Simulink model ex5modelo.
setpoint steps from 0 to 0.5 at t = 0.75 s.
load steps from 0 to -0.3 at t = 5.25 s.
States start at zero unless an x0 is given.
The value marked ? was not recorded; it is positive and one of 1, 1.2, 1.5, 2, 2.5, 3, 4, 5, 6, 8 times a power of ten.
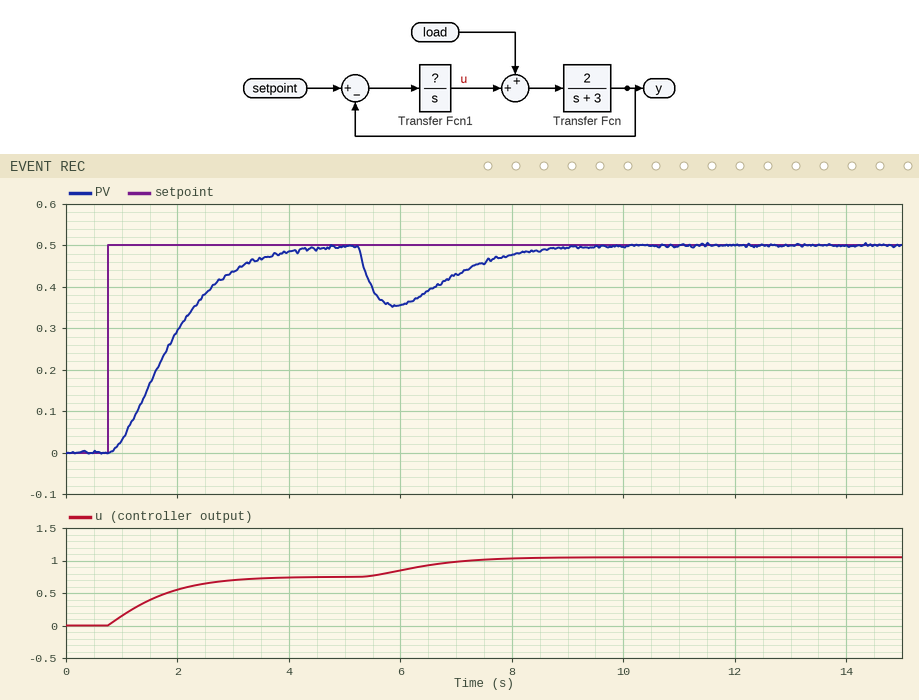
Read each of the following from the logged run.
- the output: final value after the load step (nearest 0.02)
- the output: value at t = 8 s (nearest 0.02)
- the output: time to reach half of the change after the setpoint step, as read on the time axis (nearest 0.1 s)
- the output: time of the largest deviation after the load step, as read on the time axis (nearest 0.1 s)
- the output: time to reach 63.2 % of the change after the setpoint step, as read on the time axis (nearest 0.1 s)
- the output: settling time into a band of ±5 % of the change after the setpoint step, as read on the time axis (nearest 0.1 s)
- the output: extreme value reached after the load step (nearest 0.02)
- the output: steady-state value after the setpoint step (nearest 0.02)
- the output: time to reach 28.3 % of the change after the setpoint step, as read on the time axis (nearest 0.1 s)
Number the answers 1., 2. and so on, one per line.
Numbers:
1. 0.50
2. 0.48
3. 1.8 s
4. 5.9 s
5. 2.1 s
6. 3.7 s
7. 0.36
8. 0.50
9. 1.4 s
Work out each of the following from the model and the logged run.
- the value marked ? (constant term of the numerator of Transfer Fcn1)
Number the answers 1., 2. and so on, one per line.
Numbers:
1. 1.2
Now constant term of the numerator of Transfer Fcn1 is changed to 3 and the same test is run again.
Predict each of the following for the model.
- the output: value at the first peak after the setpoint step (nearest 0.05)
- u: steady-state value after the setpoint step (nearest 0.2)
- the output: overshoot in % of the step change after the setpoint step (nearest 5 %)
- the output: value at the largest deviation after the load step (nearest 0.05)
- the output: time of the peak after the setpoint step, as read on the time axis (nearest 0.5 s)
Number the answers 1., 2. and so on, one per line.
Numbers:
1. 0.55
2. 0.8
3. 10 %
4. 0.40
5. 2.5 s
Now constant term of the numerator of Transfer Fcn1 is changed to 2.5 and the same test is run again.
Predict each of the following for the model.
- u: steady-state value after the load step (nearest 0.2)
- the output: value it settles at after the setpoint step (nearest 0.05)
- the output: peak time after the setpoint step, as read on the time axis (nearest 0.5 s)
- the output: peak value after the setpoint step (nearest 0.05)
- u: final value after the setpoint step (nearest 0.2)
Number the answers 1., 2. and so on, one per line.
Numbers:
1. 1.0
2. 0.50
3. 2.5 s
4. 0.55
5. 0.8
